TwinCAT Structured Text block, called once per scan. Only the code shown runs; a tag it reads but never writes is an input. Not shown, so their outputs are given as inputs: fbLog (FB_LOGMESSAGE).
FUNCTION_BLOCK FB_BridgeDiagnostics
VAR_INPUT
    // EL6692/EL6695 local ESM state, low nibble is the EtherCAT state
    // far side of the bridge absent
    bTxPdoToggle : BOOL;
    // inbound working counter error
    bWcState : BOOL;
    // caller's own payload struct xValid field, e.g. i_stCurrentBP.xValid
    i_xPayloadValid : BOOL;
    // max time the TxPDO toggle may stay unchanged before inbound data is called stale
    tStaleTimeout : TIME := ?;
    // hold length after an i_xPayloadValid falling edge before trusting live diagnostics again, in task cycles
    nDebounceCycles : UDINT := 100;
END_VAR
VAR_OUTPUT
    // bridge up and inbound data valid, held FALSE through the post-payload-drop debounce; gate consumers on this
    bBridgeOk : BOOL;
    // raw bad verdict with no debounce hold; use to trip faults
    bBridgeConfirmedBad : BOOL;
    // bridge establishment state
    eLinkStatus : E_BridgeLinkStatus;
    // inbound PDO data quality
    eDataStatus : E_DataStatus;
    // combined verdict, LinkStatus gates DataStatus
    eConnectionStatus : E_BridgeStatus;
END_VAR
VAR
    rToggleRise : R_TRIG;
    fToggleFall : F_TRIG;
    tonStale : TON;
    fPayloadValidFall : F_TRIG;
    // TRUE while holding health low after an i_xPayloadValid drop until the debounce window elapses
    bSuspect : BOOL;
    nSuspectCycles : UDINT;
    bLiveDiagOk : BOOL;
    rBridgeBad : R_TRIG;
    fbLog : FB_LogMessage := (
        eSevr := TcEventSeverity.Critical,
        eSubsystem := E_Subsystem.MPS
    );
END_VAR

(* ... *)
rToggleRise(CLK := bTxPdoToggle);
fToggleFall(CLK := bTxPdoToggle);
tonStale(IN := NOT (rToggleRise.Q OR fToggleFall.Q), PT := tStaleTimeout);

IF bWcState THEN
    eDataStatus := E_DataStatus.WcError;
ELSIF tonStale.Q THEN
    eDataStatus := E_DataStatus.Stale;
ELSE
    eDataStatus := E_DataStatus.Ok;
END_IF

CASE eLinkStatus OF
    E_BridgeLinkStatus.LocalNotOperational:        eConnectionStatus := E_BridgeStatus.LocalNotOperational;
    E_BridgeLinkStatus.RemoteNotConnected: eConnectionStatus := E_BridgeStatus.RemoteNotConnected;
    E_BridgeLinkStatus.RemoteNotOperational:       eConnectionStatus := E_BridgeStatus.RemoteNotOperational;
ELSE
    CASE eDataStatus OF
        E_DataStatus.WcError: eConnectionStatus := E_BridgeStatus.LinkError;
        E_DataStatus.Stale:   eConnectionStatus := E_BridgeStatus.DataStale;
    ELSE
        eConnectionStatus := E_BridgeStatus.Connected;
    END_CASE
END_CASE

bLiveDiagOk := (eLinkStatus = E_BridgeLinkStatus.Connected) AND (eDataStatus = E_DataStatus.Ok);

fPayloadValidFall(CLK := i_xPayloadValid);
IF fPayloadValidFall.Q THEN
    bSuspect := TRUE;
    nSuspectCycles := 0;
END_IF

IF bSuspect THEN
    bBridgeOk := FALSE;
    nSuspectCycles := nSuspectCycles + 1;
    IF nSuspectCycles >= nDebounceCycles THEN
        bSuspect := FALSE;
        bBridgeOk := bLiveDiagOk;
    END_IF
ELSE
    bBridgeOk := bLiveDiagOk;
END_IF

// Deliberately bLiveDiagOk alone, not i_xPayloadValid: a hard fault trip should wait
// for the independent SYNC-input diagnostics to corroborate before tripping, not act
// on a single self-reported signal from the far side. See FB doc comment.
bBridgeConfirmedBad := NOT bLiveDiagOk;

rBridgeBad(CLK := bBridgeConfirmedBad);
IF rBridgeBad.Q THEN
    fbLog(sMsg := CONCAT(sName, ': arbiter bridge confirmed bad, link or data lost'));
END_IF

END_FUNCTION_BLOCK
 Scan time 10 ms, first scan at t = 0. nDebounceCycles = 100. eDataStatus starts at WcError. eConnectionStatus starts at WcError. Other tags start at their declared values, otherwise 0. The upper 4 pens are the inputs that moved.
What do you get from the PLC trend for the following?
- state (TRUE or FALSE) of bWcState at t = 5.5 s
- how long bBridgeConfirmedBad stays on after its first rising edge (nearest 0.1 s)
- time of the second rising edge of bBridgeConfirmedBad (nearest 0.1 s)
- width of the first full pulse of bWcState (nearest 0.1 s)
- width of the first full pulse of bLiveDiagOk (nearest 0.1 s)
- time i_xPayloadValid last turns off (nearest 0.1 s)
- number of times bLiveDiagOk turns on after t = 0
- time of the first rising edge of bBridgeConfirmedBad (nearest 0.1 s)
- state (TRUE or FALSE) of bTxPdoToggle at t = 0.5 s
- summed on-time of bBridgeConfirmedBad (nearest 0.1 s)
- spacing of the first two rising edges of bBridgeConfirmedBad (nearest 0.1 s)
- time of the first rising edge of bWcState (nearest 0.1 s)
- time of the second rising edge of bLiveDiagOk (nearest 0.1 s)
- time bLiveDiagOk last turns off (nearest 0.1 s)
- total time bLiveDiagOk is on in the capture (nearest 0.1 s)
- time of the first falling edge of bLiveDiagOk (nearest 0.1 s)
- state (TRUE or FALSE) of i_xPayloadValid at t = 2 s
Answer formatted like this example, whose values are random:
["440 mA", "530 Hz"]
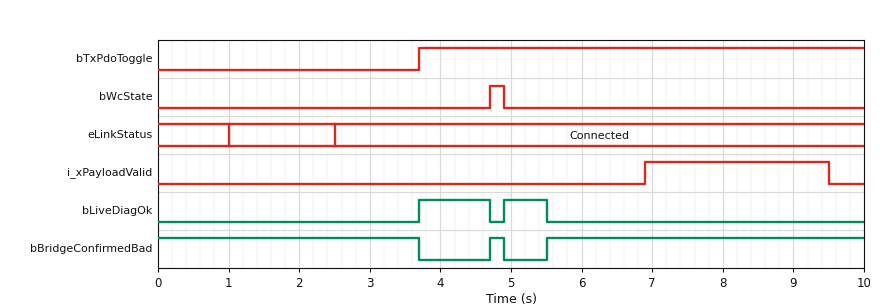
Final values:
["FALSE", "0.2 s", "5.5 s", "0.2 s", "1.0 s", "9.5 s", "2", "4.7 s", "FALSE", "8.4 s", "0.8 s", "4.7 s", "4.9 s", "5.5 s", "1.6 s", "4.7 s", "FALSE"]
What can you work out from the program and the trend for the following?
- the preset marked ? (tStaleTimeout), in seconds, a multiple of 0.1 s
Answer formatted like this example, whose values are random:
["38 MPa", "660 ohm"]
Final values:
["1.8 s"]
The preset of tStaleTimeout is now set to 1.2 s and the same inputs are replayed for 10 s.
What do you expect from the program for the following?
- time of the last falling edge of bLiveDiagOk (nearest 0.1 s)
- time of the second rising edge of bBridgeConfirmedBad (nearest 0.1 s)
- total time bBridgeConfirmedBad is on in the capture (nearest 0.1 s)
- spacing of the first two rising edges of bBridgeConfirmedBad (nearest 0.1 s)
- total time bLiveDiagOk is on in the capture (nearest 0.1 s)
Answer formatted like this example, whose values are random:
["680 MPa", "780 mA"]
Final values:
["4.9 s", "4.9 s", "9.0 s", "0.2 s", "1.0 s"]
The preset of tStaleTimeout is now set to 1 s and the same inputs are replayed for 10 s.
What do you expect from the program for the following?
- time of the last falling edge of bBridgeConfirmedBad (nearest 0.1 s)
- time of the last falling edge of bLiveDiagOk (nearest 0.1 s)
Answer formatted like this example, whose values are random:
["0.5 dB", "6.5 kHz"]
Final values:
["3.7 s", "4.7 s"]
